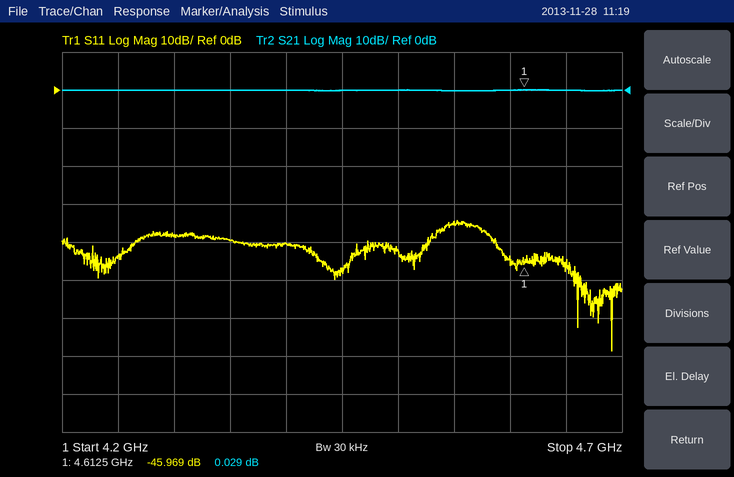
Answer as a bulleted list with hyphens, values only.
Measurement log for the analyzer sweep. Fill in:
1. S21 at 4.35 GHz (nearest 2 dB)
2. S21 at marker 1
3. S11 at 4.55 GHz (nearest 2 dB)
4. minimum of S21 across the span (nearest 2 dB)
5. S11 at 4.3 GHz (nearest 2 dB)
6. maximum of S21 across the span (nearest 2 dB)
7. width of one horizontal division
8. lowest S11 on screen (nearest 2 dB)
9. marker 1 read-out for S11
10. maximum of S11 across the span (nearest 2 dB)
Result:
- 0 dB
- 0.029 dB
- -34 dB
- 0 dB
- -38 dB
- 0 dB
- 50 MHz
- -68 dB
- -45.969 dB
- -34 dB
